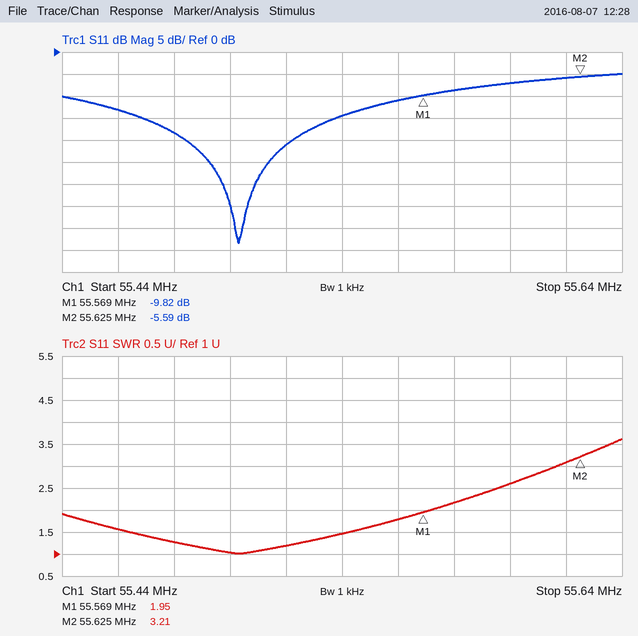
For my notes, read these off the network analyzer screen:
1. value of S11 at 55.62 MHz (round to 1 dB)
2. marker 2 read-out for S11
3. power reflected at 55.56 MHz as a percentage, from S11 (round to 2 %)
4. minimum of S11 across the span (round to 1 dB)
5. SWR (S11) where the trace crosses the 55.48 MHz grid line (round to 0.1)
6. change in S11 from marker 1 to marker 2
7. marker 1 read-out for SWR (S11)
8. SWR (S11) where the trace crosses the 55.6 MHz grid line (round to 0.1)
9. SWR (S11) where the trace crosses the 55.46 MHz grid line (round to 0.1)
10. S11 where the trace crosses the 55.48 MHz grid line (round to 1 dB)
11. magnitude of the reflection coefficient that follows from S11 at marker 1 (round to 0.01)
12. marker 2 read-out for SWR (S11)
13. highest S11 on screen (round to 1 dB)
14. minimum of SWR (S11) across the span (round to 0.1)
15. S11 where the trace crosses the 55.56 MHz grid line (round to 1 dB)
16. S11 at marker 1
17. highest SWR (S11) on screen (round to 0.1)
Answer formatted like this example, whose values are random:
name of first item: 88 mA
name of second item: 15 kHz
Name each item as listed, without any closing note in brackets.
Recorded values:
value of S11 at 55.62 MHz: -6 dB
marker 2 read-out for S11: -5.59 dB
power reflected at 55.56 MHz as a percentage, from S11: 8 %
minimum of S11 across the span: -43 dB
SWR (S11) where the trace crosses the 55.48 MHz grid line: 1.3
change in S11 from marker 1 to marker 2: 4.23 dB
marker 1 read-out for SWR: 1.95
SWR (S11) where the trace crosses the 55.6 MHz grid line: 2.6
SWR (S11) where the trace crosses the 55.46 MHz grid line: 1.6
S11 where the trace crosses the 55.48 MHz grid line: -18 dB
magnitude of the reflection coefficient that follows from S11 at marker 1: 0.32
marker 2 read-out for SWR: 3.21
highest S11 on screen: -5 dB
minimum of SWR (S11) across the span: 1.0
S11 where the trace crosses the 55.56 MHz grid line: -11 dB
S11 at marker 1: -9.82 dB
highest SWR (S11) on screen: 3.6
